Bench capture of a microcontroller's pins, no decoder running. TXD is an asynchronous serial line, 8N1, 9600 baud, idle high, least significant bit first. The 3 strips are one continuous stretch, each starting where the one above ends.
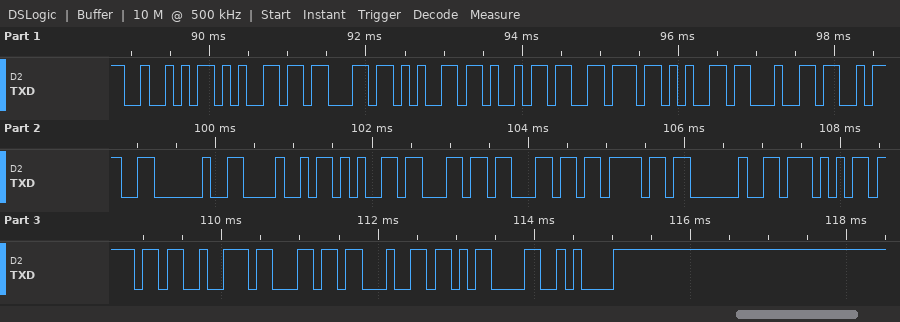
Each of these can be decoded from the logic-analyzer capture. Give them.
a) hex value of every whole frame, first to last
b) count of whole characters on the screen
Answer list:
0x52 0x65 0x63 0x65 0x69 0x76 0x65 0x64 0x3A 0x20 0x48 0x65 0x6C 0x6C 0x6F 0x20 0x57 0x6F 0x72 0x6C 0x64 0x0D 0x0A
23
